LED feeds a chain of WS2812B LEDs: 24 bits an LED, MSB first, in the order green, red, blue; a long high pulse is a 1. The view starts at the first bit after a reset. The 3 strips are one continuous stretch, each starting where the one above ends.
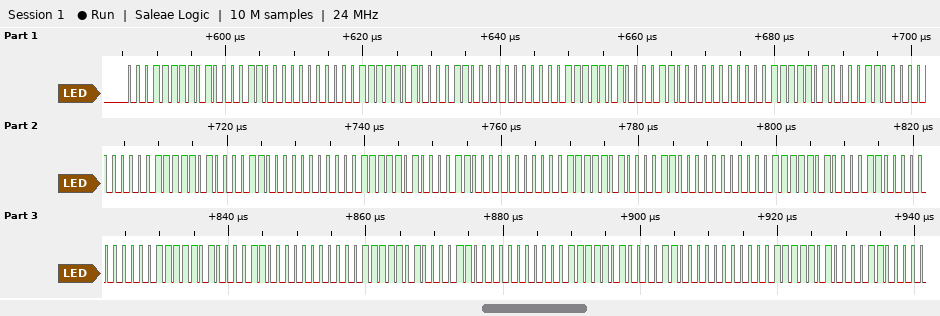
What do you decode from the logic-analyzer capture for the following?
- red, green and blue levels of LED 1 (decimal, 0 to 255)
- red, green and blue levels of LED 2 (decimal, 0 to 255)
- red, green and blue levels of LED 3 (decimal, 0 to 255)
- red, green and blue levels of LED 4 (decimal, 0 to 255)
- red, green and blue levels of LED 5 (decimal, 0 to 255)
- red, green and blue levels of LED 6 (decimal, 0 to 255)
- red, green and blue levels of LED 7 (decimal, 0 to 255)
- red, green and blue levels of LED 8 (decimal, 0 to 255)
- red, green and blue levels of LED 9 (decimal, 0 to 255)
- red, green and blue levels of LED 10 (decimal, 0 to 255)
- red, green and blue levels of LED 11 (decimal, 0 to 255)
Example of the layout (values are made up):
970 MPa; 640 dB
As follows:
67, 31, 0; 67, 31, 0; 67, 31, 0; 67, 31, 0; 67, 31, 0; 67, 31, 0; 67, 31, 0; 67, 31, 0; 67, 31, 0; 67, 31, 0; 67, 31, 0
